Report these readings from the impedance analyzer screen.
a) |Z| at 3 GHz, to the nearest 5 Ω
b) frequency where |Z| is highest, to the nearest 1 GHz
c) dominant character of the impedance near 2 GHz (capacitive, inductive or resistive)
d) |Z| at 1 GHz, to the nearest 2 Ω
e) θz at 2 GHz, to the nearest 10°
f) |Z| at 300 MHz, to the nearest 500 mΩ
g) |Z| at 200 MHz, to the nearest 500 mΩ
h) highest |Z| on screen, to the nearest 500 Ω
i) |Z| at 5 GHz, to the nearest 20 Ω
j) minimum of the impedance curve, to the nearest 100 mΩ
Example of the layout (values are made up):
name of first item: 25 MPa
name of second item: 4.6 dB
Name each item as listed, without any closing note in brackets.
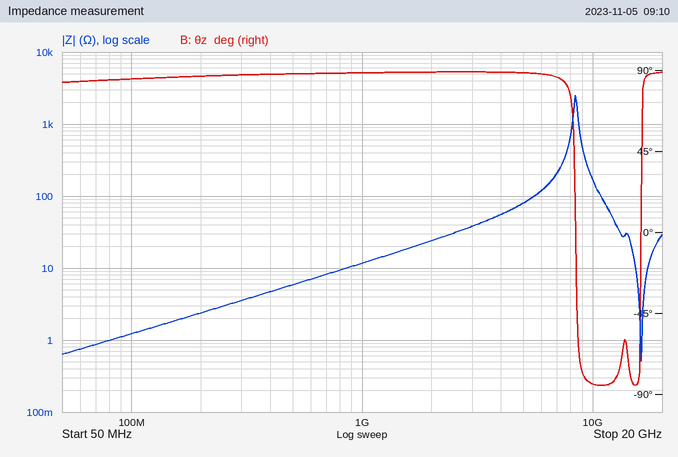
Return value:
|Z| at 3 GHz, to the nearest 5 Ω: 40 Ω
frequency where |Z| is highest, to the nearest 1 GHz: 8 GHz
dominant character of the impedance near 2 GHz: inductive
|Z| at 1 GHz, to the nearest 2 Ω: 12 Ω
θz at 2 GHz, to the nearest 10°: 90°
|Z| at 300 MHz, to the nearest 500 mΩ: 3.5 Ω
|Z| at 200 MHz, to the nearest 500 mΩ: 2.5 Ω
highest |Z| on screen, to the nearest 500 Ω: 2.5 kΩ
|Z| at 5 GHz, to the nearest 20 Ω: 80 Ω
minimum of the impedance curve, to the nearest 100 mΩ: 500 mΩ
